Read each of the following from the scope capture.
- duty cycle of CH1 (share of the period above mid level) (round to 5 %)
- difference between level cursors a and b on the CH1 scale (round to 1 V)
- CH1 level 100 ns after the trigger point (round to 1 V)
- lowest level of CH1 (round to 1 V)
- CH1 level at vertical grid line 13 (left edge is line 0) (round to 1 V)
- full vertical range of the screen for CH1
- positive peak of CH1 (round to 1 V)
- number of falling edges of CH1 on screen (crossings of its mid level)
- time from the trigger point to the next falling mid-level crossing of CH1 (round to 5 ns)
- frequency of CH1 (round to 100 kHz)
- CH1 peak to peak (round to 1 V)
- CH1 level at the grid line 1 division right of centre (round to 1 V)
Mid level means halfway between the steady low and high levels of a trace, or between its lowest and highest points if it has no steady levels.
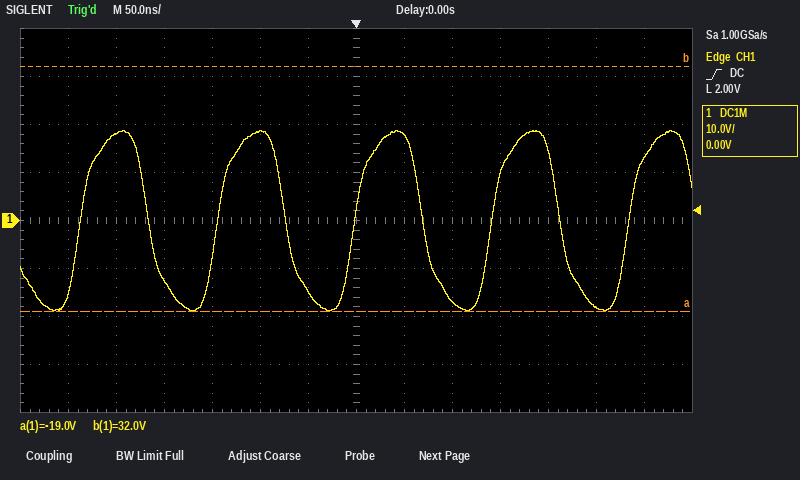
50 %
51 V
-17 V
-19 V
13 V
80 V
19 V
4
70 ns
7.0 MHz
38 V
18 V
